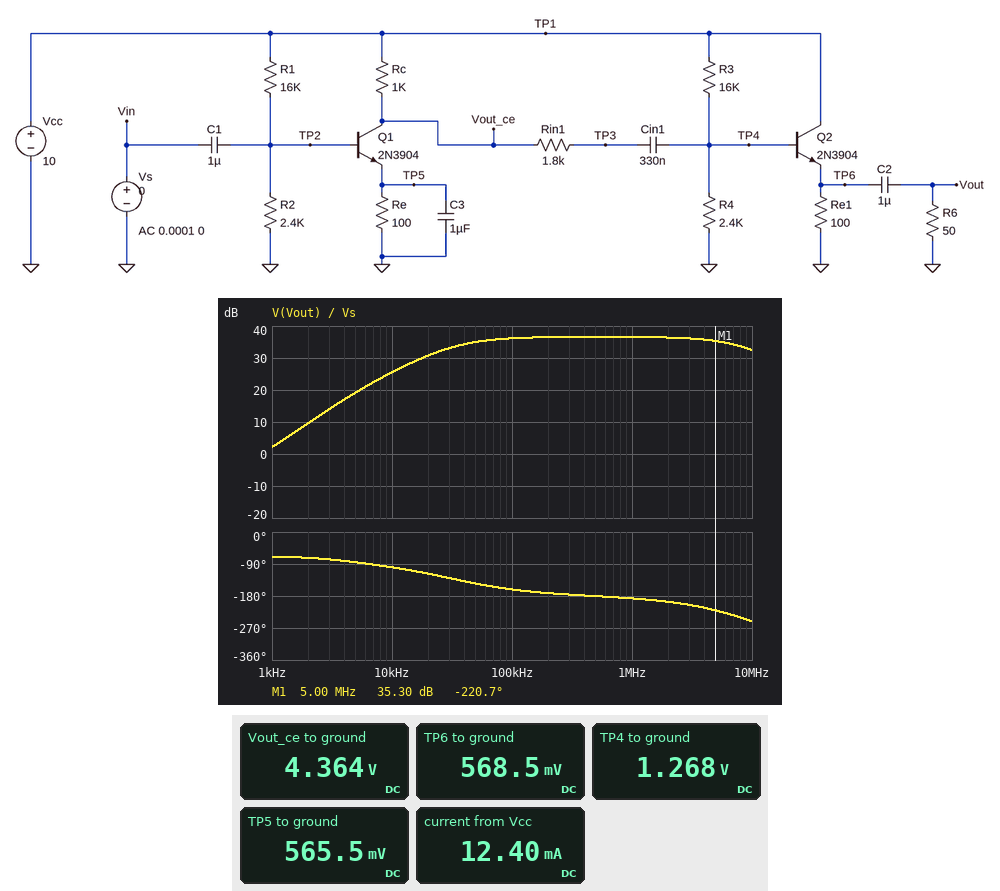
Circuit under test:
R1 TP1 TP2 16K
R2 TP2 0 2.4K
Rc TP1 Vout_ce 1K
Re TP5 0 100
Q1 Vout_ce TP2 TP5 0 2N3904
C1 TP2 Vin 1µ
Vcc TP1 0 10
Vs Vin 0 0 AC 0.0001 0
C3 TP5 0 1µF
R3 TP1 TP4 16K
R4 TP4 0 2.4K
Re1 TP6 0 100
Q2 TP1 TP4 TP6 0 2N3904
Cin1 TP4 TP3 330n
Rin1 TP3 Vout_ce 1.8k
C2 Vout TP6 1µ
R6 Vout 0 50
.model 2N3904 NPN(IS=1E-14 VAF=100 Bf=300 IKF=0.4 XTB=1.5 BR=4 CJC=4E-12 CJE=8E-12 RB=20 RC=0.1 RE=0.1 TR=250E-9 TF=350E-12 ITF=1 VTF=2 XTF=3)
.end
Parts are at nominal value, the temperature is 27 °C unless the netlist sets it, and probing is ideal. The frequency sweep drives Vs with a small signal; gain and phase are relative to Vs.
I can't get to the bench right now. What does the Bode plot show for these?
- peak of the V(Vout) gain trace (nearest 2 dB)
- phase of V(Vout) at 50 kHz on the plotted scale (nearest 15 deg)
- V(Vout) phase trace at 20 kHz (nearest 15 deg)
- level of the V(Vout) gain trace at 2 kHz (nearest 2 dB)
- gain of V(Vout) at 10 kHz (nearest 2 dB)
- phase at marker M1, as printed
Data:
36 dB
-150 deg
-120 deg
10 dB
26 dB
-220.7 deg
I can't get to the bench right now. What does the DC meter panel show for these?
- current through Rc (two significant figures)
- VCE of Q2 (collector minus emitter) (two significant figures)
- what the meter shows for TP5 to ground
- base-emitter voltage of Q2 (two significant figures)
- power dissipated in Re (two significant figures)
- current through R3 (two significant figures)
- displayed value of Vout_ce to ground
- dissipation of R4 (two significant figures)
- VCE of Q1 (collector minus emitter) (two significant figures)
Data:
5.6 mA
9.4 V
565.5 mV
700 mV
3.2 mW
550 µA
4.364 V
670 µW
3.8 V
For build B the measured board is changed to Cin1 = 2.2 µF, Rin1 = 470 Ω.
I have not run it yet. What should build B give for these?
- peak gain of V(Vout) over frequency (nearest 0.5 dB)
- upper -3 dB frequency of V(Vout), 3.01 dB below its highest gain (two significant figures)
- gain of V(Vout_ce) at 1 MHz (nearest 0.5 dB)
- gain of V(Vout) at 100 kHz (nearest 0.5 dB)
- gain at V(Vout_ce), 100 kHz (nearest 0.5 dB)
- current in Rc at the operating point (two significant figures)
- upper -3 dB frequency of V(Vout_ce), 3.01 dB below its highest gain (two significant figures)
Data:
39.5 dB
9.4 MHz
43.0 dB
39.0 dB
42.5 dB
5.6 mA
10 MHz
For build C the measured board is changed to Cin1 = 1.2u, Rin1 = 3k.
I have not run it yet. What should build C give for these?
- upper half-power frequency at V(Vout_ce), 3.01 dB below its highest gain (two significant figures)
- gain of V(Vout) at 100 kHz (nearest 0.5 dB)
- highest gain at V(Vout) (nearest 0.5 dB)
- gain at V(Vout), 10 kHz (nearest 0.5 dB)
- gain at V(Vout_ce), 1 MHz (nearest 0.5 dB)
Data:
13 MHz
34.0 dB
34.5 dB
23.5 dB
44.5 dB
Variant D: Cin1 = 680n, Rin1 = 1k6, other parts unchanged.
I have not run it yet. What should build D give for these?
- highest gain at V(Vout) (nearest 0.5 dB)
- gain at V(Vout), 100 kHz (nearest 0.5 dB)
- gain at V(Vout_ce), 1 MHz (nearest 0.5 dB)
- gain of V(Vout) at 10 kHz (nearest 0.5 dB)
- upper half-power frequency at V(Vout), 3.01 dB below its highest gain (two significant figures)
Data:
37.0 dB
36.5 dB
43.5 dB
26.0 dB
8.3 MHz
